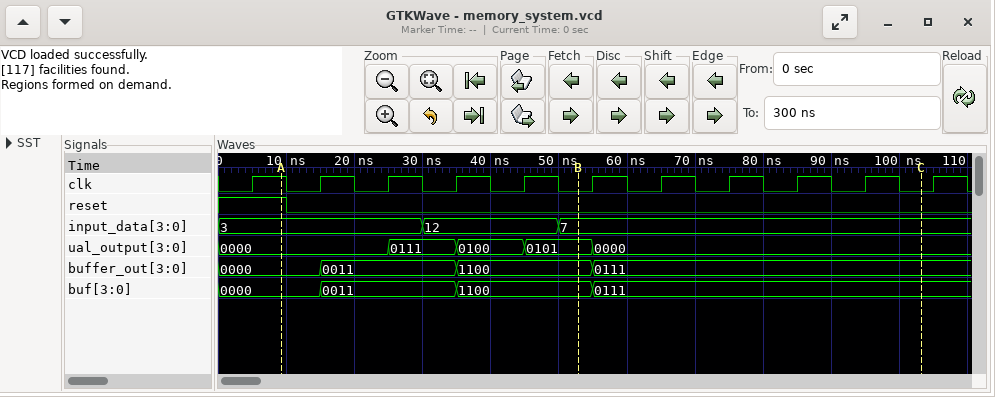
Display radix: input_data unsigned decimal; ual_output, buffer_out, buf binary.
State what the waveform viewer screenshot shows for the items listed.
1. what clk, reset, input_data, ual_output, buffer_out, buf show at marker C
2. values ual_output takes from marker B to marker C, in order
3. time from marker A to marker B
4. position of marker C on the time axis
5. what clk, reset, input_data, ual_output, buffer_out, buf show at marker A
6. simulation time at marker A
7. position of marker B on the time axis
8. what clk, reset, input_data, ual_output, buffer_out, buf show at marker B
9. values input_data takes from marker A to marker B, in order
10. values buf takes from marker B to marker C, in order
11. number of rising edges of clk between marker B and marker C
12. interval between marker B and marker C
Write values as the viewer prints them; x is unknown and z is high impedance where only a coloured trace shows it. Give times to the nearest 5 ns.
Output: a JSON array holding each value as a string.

["clk=0, reset=0, input_data=7, ual_output=0000, buffer_out=0111, buf=0111", "0101, 0000", "45 ns", "105 ns", "clk=1, reset=1, input_data=3, ual_output=0000, buffer_out=0000, buf=0000", "10 ns", "55 ns", "clk=0, reset=0, input_data=7, ual_output=0101, buffer_out=1100, buf=1100", "3, 12, 7", "1100, 0111", "5", "50 ns"]
